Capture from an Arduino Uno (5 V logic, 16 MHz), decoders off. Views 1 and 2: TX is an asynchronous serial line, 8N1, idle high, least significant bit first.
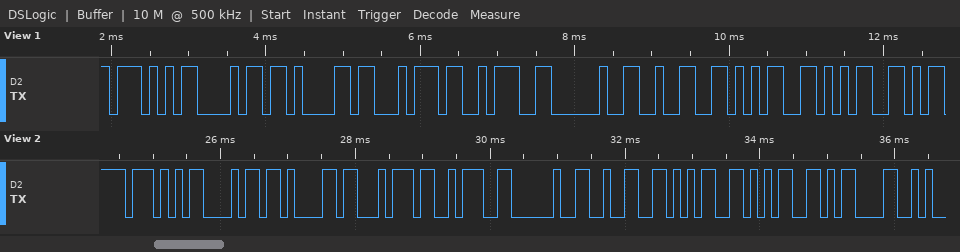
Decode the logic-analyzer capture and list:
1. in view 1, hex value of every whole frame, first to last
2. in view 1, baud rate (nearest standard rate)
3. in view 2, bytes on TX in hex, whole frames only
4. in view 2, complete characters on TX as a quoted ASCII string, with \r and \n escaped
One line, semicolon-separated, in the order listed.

0x57 0x68 0x61 0x74 0x3A 0x20 0x32 0x35 0x35; 9600 baud; 0x57 0x68 0x61 0x74 0x3A 0x20 0x32 0x35 0x35 0x0D; "What: 255\r"
